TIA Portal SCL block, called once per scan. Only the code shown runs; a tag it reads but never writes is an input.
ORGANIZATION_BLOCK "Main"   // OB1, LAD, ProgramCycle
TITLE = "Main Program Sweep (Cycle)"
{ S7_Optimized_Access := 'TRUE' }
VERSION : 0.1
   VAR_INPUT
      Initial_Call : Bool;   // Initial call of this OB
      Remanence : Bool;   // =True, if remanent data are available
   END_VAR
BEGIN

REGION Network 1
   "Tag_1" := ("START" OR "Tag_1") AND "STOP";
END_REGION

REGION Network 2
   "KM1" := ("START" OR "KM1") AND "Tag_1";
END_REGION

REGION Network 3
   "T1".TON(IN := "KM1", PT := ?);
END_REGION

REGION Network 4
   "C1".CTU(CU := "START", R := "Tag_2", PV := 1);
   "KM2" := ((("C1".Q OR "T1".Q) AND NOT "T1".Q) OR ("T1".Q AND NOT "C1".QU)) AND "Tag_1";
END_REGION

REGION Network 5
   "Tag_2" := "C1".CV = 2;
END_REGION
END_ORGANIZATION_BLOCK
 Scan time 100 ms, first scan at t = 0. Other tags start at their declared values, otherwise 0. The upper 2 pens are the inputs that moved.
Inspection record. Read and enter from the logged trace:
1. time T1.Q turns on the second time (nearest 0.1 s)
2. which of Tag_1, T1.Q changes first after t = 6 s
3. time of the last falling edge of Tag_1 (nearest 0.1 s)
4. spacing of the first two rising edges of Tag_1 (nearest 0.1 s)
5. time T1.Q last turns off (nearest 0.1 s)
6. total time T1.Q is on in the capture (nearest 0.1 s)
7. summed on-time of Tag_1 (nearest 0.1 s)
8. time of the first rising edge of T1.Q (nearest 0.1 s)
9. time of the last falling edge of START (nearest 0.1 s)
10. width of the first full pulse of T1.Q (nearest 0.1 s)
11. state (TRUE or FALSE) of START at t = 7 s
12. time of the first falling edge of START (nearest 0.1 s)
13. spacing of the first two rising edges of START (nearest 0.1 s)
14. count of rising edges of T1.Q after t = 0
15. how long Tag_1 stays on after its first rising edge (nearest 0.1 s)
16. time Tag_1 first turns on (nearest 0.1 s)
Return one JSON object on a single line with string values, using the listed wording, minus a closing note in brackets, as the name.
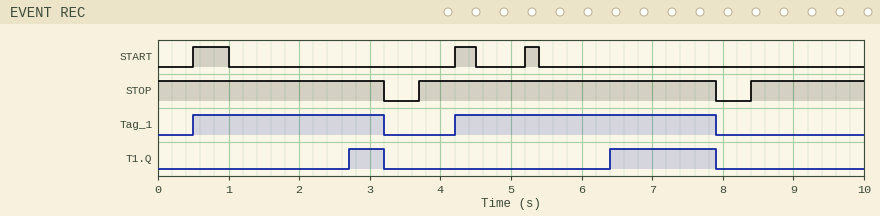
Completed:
{"time T1.Q turns on the second time": "6.4 s", "which of Tag_1, T1.Q changes first after t = 6 s": "T1.Q", "time of the last falling edge of Tag_1": "7.9 s", "spacing of the first two rising edges of Tag_1": "3.7 s", "time T1.Q last turns off": "7.9 s", "total time T1.Q is on in the capture": "2.0 s", "summed on-time of Tag_1": "6.4 s", "time of the first rising edge of T1.Q": "2.7 s", "time of the last falling edge of START": "5.4 s", "width of the first full pulse of T1.Q": "0.5 s", "state (TRUE or FALSE) of START at t = 7 s": "FALSE", "time of the first falling edge of START": "1.0 s", "spacing of the first two rising edges of START": "3.7 s", "count of rising edges of T1.Q after t = 0": "2", "how long Tag_1 stays on after its first rising edge": "2.7 s", "time Tag_1 first turns on": "0.5 s"}
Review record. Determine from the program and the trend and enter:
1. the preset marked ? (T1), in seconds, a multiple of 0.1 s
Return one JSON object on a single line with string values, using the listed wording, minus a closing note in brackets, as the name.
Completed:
{"the preset marked ? (T1), in seconds, a multiple of 0.1 s": "2.2 s"}
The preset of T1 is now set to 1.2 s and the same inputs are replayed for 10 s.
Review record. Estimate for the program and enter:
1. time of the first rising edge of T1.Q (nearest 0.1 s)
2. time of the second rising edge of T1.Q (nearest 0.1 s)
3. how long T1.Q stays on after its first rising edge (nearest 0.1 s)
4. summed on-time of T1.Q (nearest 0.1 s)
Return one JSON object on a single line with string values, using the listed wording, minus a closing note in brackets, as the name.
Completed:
{"time of the first rising edge of T1.Q": "1.7 s", "time of the second rising edge of T1.Q": "5.4 s", "how long T1.Q stays on after its first rising edge": "1.5 s", "summed on-time of T1.Q": "4.0 s"}
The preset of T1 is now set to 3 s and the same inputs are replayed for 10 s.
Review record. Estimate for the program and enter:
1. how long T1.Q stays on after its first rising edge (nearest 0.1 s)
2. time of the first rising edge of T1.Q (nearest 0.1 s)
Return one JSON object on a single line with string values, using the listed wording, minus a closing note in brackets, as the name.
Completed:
{"how long T1.Q stays on after its first rising edge": "0.7 s", "time of the first rising edge of T1.Q": "7.2 s"}
